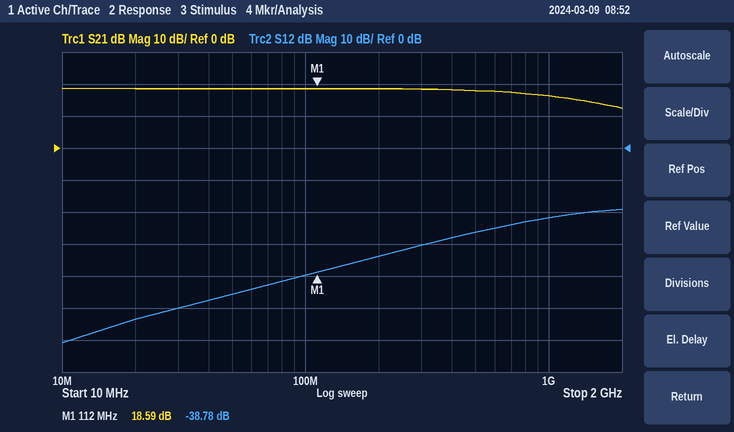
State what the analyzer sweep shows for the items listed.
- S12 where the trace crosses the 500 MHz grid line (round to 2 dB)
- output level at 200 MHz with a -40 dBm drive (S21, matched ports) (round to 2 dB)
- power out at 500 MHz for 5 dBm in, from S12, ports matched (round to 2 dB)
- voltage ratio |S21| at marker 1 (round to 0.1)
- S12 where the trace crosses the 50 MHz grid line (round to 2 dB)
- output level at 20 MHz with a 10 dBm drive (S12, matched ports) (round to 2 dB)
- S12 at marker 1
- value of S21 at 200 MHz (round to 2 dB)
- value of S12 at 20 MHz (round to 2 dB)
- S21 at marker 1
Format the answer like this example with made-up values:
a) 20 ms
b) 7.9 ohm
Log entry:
a) -26 dB
b) -22 dBm
c) -22 dBm
d) 8.5
e) -46 dB
f) -44 dBm
g) -38.78 dB
h) 18 dB
i) -54 dB
j) 18.59 dB
